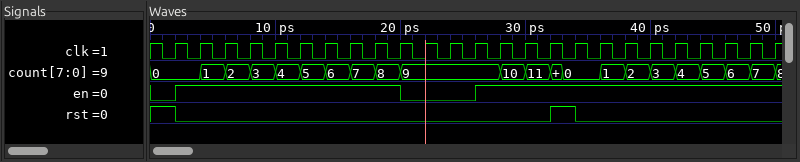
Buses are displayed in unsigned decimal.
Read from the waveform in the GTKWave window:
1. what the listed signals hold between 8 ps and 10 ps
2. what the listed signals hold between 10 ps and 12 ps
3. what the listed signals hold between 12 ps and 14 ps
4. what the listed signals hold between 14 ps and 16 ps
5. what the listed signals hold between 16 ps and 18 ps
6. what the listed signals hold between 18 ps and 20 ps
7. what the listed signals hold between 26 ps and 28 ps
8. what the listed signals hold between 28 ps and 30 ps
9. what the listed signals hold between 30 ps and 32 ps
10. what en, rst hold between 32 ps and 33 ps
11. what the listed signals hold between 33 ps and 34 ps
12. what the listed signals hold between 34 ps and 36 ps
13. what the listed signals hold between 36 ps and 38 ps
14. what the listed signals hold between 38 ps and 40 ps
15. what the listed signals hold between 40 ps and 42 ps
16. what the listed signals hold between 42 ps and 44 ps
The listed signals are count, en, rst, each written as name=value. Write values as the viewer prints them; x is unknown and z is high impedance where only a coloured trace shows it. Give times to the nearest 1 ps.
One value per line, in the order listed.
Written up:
count=3, en=1, rst=0
count=4, en=1, rst=0
count=5, en=1, rst=0
count=6, en=1, rst=0
count=7, en=1, rst=0
count=8, en=1, rst=0
count=9, en=1, rst=0
count=10, en=1, rst=0
count=11, en=1, rst=0
en=1, rst=1
count=0, en=1, rst=1
count=0, en=1, rst=0
count=1, en=1, rst=0
count=2, en=1, rst=0
count=3, en=1, rst=0
count=4, en=1, rst=0
